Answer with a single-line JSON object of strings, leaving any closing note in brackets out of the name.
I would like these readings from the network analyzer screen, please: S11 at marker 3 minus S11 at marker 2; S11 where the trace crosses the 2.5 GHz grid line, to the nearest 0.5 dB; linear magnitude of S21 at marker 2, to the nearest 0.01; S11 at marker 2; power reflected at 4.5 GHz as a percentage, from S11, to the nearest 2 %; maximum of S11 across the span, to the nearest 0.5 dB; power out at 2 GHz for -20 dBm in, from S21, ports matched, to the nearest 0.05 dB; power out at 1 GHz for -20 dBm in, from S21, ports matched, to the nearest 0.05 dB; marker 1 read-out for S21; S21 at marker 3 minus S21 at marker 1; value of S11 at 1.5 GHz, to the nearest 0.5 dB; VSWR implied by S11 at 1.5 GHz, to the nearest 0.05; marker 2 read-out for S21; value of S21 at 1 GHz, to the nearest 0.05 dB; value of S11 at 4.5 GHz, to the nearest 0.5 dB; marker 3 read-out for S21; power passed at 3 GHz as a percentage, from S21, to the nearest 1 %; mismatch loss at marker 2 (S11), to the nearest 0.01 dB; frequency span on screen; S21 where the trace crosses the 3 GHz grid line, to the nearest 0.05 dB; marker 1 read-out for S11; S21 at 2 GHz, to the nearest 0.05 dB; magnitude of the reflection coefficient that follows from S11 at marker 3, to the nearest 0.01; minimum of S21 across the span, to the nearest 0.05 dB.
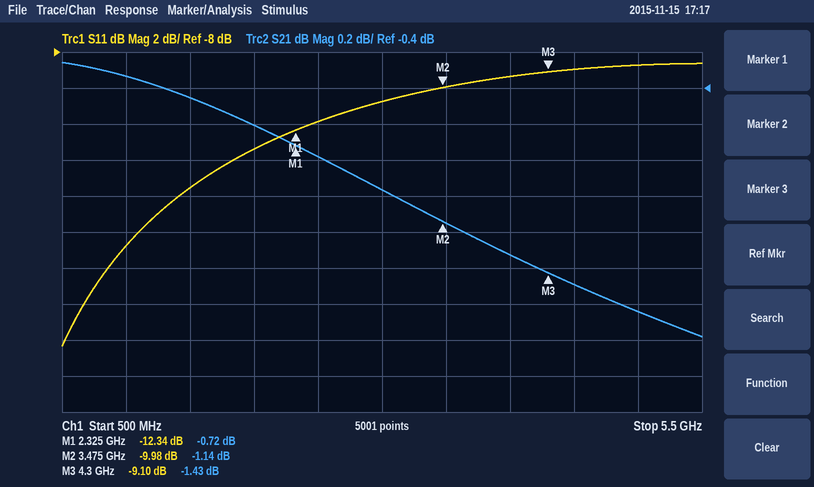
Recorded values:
{"S11 at marker 3 minus S11 at marker 2": "0.88 dB", "S11 where the trace crosses the 2.5 GHz grid line, to the nearest 0.5 dB": "-12.0 dB", "linear magnitude of S21 at marker 2, to the nearest 0.01": "0.88", "S11 at marker 2": "-9.98 dB", "power reflected at 4.5 GHz as a percentage, from S11, to the nearest 2 %": "12 %", "maximum of S11 across the span, to the nearest 0.5 dB": "-8.5 dB", "power out at 2 GHz for -20 dBm in, from S21, ports matched, to the nearest 0.05 dB": "-20.60 dBm", "power out at 1 GHz for -20 dBm in, from S21, ports matched, to the nearest 0.05 dB": "-20.35 dBm", "marker 1 read-out for S21": "-0.72 dB", "S21 at marker 3 minus S21 at marker 1": "-0.71 dB", "value of S11 at 1.5 GHz, to the nearest 0.5 dB": "-15.5 dB", "VSWR implied by S11 at 1.5 GHz, to the nearest 0.05": "1.40", "marker 2 read-out for S21": "-1.14 dB", "value of S21 at 1 GHz, to the nearest 0.05 dB": "-0.35 dB", "value of S11 at 4.5 GHz, to the nearest 0.5 dB": "-9.0 dB", "marker 3 read-out for S21": "-1.43 dB", "power passed at 3 GHz as a percentage, from S21, to the nearest 1 %": "80 %", "mismatch loss at marker 2 (S11), to the nearest 0.01 dB": "0.46 dB", "frequency span on screen": "5 GHz", "S21 where the trace crosses the 3 GHz grid line, to the nearest 0.05 dB": "-0.95 dB", "marker 1 read-out for S11": "-12.34 dB", "S21 at 2 GHz, to the nearest 0.05 dB": "-0.60 dB", "magnitude of the reflection coefficient that follows from S11 at marker 3, to the nearest 0.01": "0.35", "minimum of S21 across the span, to the nearest 0.05 dB": "-1.80 dB"}
